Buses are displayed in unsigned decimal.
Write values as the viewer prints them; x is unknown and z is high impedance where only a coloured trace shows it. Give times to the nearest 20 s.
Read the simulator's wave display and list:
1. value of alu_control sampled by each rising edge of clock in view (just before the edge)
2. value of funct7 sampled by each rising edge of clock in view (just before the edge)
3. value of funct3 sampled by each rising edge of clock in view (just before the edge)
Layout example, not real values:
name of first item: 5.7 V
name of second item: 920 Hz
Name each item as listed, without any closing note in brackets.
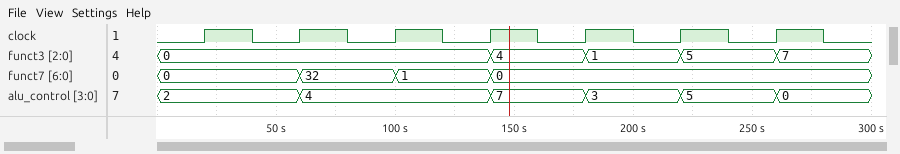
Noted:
value of alu_control sampled by each rising edge of clock in view: 2, 2, 4, 4, 7, 3, 5
value of funct7 sampled by each rising edge of clock in view: 0, 0, 32, 1, 0, 0, 0
value of funct3 sampled by each rising edge of clock in view: 0, 0, 0, 0, 4, 1, 5
